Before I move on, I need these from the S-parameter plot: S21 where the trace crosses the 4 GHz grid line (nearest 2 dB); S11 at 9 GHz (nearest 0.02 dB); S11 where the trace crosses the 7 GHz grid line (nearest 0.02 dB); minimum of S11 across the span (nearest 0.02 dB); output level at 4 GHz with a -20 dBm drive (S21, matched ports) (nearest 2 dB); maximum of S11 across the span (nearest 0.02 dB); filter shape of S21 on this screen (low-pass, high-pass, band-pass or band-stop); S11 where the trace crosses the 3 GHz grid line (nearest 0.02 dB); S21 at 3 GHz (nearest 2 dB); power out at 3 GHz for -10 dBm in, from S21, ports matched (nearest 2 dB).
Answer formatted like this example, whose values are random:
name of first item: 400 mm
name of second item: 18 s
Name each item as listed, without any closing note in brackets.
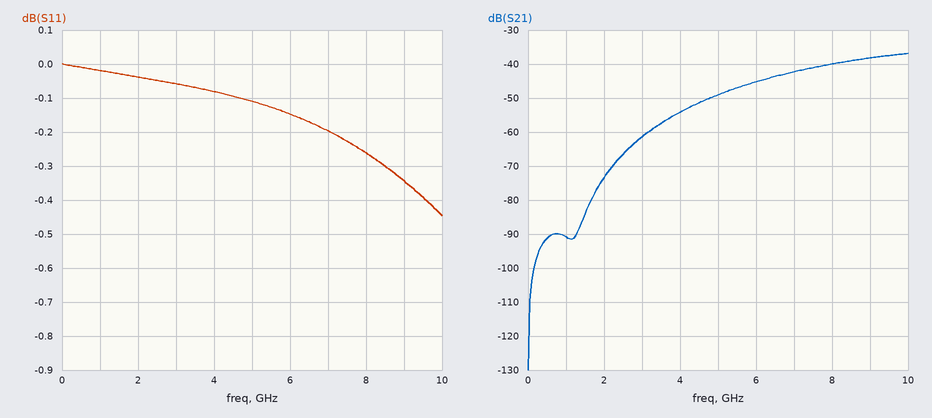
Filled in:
S21 where the trace crosses the 4 GHz grid line: -54 dB
S11 at 9 GHz: -0.34 dB
S11 where the trace crosses the 7 GHz grid line: -0.20 dB
minimum of S11 across the span: -0.44 dB
output level at 4 GHz with a -20 dBm drive (S21, matched ports): -74 dBm
maximum of S11 across the span: 0.00 dB
filter shape of S21 on this screen: high-pass
S11 where the trace crosses the 3 GHz grid line: -0.06 dB
S21 at 3 GHz: -62 dB
power out at 3 GHz for -10 dBm in, from S21, ports matched: -72 dBm
